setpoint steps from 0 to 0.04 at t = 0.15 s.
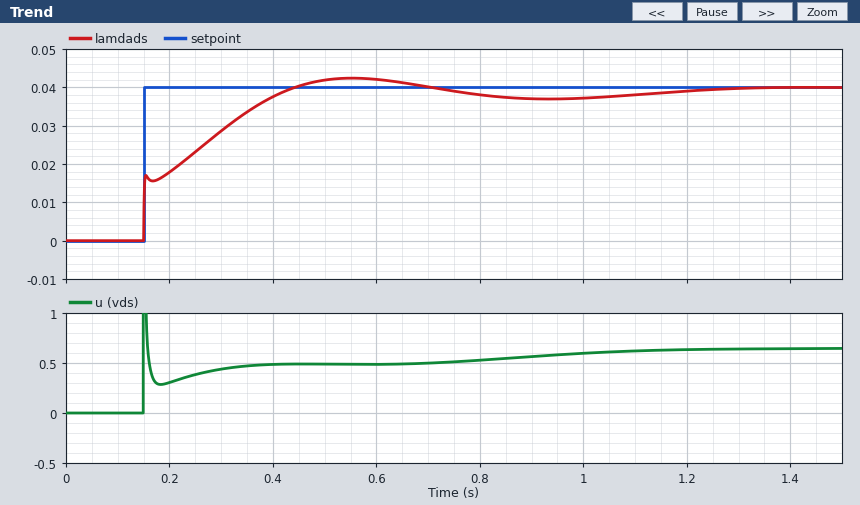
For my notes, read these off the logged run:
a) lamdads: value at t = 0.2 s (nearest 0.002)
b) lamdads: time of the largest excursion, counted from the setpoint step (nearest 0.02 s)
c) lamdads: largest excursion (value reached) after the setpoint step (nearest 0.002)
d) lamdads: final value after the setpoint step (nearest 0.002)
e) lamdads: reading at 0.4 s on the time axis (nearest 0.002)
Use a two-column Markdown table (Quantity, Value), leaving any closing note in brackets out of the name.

| Quantity | Value |
|---|---|
| lamdads: value at t = 0.2 s | 0.018 |
| lamdads: time of the largest excursion, counted from the setpoint step | 0.40 s |
| lamdads: largest excursion (value reached) after the setpoint step | 0.042 |
| lamdads: final value after the setpoint step | 0.040 |
| lamdads: reading at 0.4 s on the time axis | 0.038 |
